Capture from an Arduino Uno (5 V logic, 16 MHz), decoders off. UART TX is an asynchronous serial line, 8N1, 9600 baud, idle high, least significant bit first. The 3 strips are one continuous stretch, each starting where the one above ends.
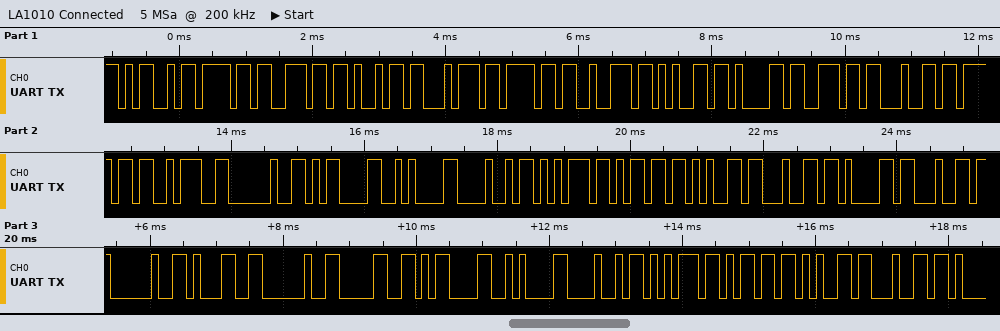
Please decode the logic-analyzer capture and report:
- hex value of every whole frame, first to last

4D 6F 6E 69 74 6F 72 65 61 6E 64 6F 3A 20 0D 0A 48 75 6D 65 64 61 64 20 31 20 30 0D 0A 48 75 6D 65 64
